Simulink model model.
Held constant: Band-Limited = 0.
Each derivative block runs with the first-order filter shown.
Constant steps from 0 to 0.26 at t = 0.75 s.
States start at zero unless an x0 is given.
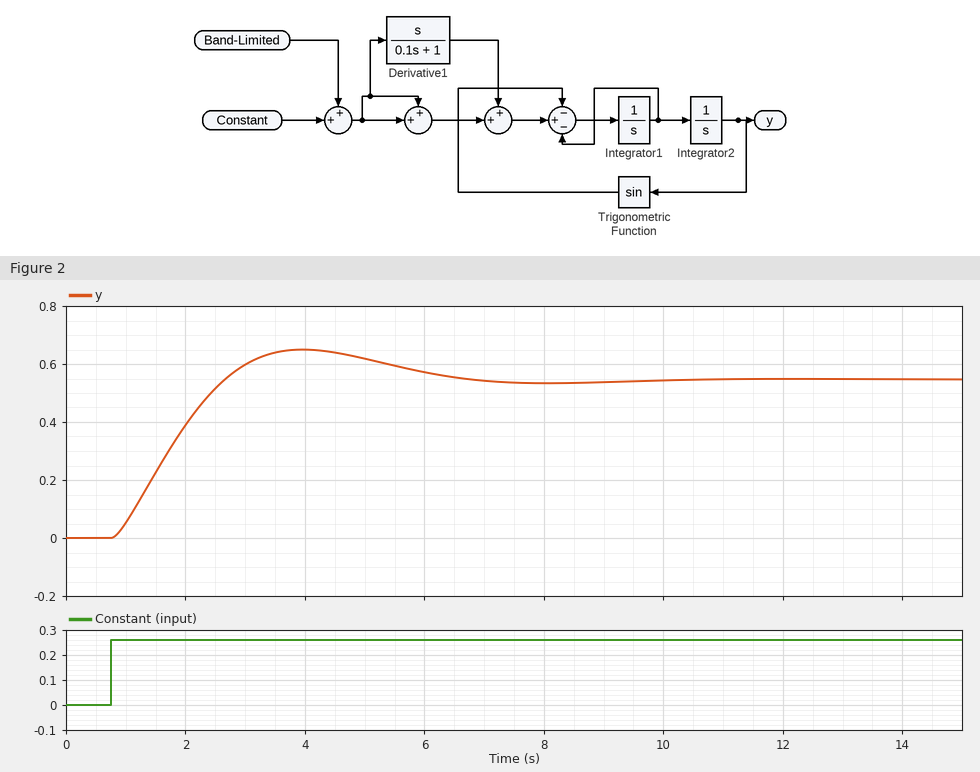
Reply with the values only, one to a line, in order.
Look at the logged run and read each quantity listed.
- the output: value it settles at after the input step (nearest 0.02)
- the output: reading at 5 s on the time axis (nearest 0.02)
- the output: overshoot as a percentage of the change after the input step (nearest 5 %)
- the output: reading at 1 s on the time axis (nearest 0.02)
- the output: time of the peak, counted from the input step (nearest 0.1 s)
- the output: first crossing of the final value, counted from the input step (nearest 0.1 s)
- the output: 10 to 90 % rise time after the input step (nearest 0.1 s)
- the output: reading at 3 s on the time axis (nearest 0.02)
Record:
0.54
0.62
20 %
0.06
3.2 s
1.9 s
1.4 s
0.60
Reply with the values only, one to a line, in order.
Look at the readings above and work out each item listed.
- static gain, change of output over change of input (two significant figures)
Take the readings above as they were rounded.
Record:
2.1
